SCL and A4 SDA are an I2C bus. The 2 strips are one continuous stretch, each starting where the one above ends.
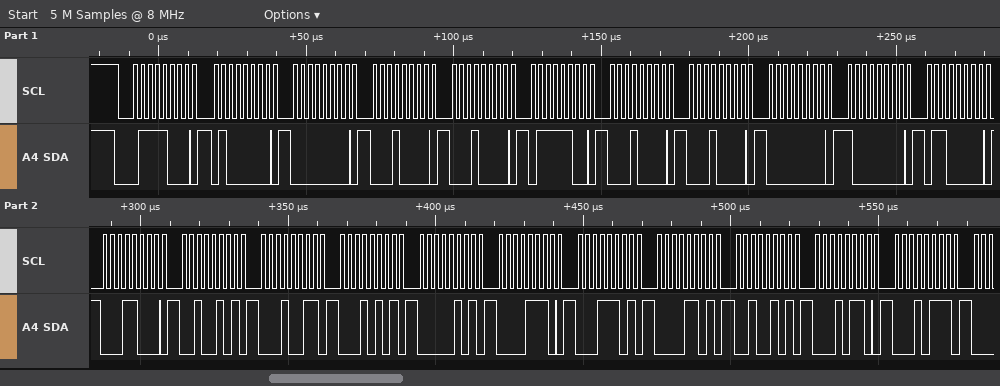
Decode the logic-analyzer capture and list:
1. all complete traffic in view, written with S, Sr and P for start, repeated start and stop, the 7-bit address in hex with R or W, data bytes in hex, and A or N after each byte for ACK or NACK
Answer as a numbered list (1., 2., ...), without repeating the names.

1. S 3CW A 40 A 00 A 10 A 10 A 7C A 10 A 10 A 00 A 80 A 60 A 18 A 25 A 13 A 15 A 05 A 0E A 1D A 0D A 25 A 16 A 17 A
